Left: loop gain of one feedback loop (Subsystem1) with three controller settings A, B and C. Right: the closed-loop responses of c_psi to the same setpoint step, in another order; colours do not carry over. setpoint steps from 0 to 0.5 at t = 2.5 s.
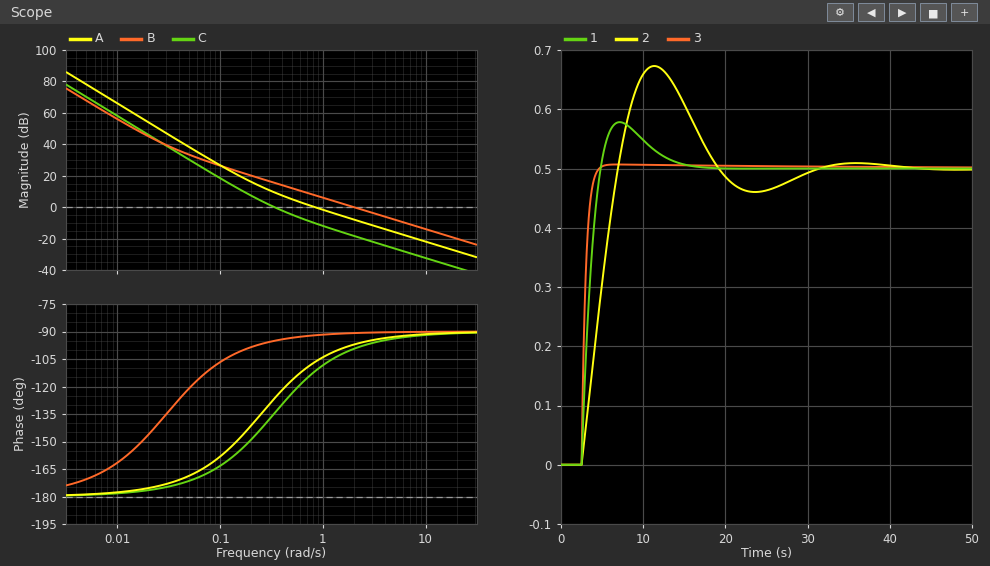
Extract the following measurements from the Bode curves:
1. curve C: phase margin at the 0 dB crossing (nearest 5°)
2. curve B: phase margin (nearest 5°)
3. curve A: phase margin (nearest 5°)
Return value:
45°
90°
75°
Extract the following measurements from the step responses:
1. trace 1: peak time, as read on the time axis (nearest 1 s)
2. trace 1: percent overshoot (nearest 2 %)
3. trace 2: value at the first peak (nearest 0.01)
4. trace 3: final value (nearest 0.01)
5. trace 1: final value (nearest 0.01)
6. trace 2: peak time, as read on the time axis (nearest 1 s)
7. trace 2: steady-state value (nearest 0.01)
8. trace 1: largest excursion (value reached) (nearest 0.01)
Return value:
7 s
16 %
0.67
0.50
0.50
11 s
0.50
0.58
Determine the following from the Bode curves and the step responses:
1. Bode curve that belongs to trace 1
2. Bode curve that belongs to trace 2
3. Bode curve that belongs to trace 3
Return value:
A
C
B
